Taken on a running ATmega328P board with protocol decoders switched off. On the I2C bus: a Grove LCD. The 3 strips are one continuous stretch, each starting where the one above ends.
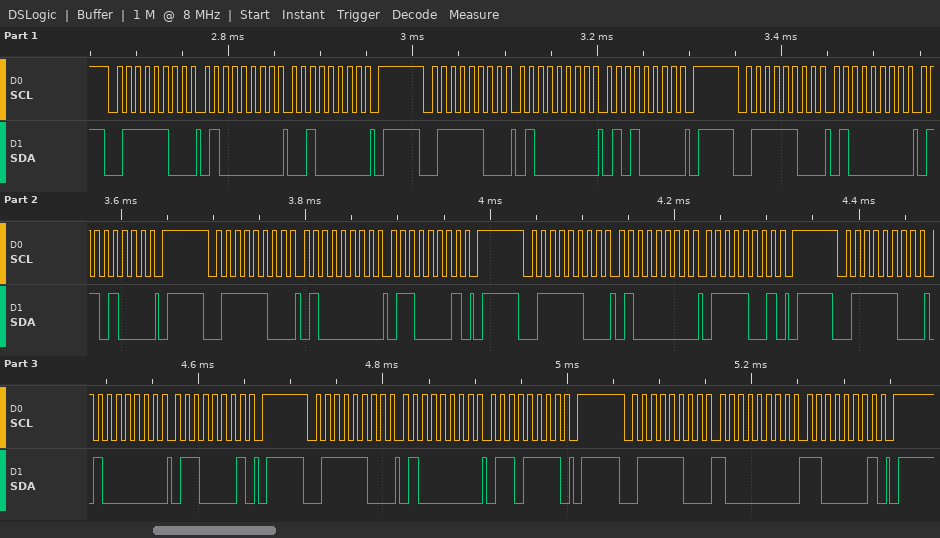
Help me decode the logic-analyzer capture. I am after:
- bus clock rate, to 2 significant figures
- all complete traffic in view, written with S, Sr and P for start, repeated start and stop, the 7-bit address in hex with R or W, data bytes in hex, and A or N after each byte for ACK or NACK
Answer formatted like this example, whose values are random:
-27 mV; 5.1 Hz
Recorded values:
100 kHz; S 3EW A 40 A 20 A P S 3EW A 40 A 50 A P S 3EW A 40 A 68 A P S 3EW A 40 A 61 A P S 3EW A 40 A 79 A P S 3EW A 40 A 61 A P S 3EW A 40 A 6F A P S 3EW A 80 A C1 A P
